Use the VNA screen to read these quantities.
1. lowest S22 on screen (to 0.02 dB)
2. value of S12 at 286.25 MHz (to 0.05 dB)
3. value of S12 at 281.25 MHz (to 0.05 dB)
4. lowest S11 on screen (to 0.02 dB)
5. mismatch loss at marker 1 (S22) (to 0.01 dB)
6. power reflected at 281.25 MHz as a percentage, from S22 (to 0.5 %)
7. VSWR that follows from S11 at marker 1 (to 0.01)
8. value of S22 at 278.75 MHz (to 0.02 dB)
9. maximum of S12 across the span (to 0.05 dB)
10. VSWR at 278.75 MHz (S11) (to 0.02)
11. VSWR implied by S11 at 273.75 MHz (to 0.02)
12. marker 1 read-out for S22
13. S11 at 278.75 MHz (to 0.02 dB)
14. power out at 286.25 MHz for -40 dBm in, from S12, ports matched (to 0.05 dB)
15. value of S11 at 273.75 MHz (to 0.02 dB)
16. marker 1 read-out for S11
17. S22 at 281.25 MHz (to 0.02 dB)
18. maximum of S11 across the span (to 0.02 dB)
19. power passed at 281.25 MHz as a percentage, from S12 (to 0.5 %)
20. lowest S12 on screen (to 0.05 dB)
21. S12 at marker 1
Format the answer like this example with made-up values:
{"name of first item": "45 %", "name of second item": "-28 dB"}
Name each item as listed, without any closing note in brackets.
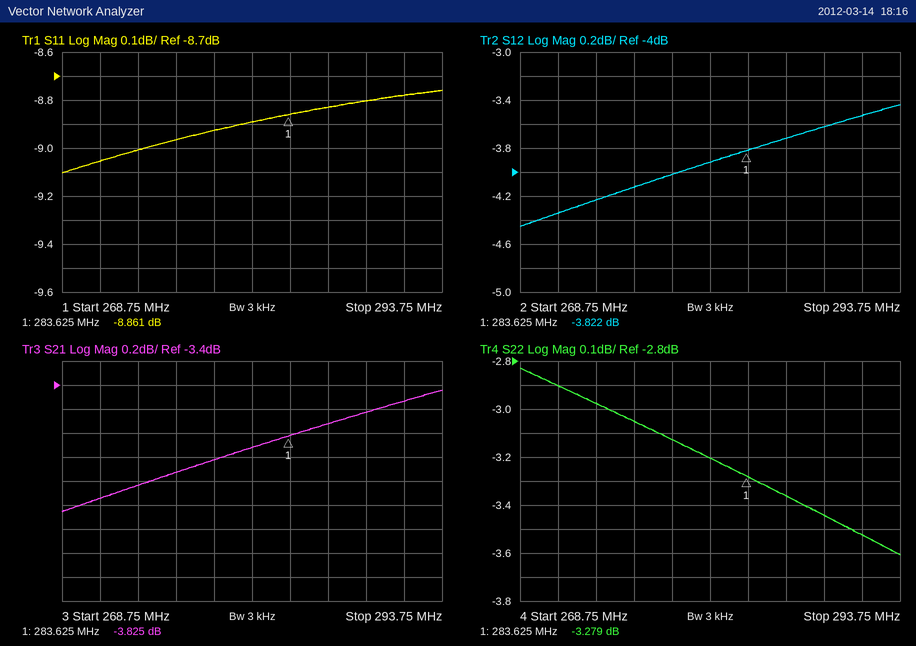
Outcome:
{"lowest S22 on screen": "-3.60 dB", "value of S12 at 286.25 MHz": "-3.70 dB", "value of S12 at 281.25 MHz": "-3.90 dB", "lowest S11 on screen": "-9.10 dB", "mismatch loss at marker 1 (S22)": "2.76 dB", "power reflected at 281.25 MHz as a percentage, from S22": "48.0 %", "VSWR that follows from S11 at marker 1": "2.13", "value of S22 at 278.75 MHz": "-3.12 dB", "maximum of S12 across the span": "-3.45 dB", "VSWR at 278.75 MHz (S11)": "2.12", "VSWR implied by S11 at 273.75 MHz": "2.10", "marker 1 read-out for S22": "-3.279 dB", "S11 at 278.75 MHz": "-8.92 dB", "power out at 286.25 MHz for -40 dBm in, from S12, ports matched": "-43.70 dBm", "value of S11 at 273.75 MHz": "-9.00 dB", "marker 1 read-out for S11": "-8.861 dB", "S22 at 281.25 MHz": "-3.20 dB", "maximum of S11 across the span": "-8.76 dB", "power passed at 281.25 MHz as a percentage, from S12": "40.5 %", "lowest S12 on screen": "-4.45 dB", "S12 at marker 1": "-3.822 dB"}
